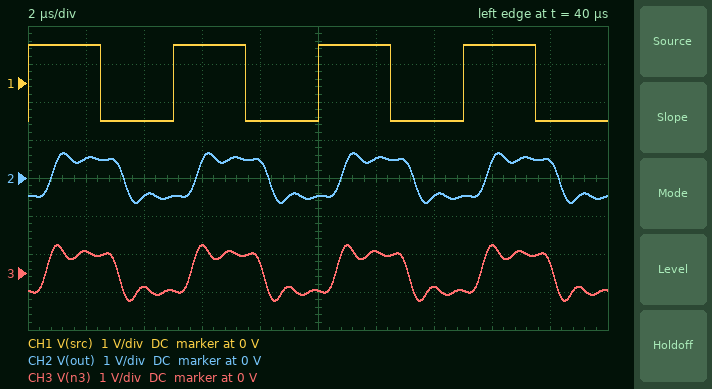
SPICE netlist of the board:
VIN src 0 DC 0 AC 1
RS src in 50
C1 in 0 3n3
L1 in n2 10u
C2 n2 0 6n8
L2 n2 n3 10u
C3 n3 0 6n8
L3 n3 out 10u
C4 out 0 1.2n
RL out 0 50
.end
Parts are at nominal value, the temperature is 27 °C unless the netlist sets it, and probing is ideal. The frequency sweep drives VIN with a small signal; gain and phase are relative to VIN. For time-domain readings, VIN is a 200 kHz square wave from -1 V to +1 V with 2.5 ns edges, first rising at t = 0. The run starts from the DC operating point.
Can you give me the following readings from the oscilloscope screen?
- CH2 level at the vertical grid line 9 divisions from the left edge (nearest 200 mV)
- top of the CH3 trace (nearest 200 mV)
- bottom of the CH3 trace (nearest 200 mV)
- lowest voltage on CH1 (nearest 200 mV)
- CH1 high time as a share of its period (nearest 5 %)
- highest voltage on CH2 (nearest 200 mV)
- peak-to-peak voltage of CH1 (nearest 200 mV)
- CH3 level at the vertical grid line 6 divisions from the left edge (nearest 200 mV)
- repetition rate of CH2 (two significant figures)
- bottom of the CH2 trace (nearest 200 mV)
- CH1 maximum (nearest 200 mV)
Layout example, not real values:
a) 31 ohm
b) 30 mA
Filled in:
a) 400 mV
b) 800 mV
c) -800 mV
d) -1.0 V
e) 50 %
f) 600 mV
g) 2.0 V
h) 600 mV
i) 200 kHz
j) -600 mV
k) 1.0 V
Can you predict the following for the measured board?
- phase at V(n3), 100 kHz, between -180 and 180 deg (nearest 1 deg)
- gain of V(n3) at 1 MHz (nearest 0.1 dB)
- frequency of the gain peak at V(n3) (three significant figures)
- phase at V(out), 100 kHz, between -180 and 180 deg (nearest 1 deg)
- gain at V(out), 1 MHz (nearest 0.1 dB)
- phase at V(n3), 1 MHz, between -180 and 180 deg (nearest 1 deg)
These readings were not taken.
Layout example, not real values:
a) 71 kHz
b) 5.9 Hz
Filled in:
a) -20 deg
b) -3.6 dB
c) 1.03 MHz
d) -27 deg
e) -6.3 dB
f) 120 deg
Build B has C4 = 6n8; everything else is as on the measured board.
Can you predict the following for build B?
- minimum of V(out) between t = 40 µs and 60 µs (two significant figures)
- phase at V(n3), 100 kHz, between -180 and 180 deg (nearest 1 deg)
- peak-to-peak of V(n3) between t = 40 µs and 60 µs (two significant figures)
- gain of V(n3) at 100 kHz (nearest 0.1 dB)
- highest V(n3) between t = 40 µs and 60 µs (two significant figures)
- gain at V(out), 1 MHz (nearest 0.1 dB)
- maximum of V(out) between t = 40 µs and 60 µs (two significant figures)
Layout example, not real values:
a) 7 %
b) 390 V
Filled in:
a) -640 mV
b) -24 deg
c) 1.3 V
d) -6.3 dB
e) 650 mV
f) -7.7 dB
g) 640 mV
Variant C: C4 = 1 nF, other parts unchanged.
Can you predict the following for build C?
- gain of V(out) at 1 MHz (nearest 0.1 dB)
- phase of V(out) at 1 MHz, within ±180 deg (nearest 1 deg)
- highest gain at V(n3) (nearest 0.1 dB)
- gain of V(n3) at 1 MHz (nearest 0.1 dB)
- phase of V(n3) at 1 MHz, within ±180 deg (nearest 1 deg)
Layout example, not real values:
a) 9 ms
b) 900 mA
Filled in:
a) -6.4 dB
b) 55 deg
c) -3.4 dB
d) -3.5 dB
e) 119 deg
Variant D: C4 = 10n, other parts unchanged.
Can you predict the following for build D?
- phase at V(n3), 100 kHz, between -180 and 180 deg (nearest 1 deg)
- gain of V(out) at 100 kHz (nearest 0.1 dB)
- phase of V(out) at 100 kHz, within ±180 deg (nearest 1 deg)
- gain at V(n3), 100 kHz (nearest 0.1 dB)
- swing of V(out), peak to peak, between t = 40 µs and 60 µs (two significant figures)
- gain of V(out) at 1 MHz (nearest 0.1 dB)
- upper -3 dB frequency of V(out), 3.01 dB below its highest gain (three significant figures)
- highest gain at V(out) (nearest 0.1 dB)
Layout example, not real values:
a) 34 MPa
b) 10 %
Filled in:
a) -27 deg
b) -6.2 dB
c) -34 deg
d) -6.5 dB
e) 1.2 V
f) -10.0 dB
g) 868 kHz
h) -6.0 dB
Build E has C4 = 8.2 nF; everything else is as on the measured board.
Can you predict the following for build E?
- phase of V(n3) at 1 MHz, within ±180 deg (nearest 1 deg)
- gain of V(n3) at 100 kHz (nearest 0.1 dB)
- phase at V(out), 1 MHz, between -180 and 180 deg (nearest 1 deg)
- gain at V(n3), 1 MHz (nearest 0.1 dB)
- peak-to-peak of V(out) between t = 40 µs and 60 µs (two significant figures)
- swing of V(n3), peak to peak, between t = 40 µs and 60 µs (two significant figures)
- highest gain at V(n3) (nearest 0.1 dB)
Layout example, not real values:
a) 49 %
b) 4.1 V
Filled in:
a) 146 deg
b) -6.4 dB
c) -4 deg
d) -0.5 dB
e) 1.2 V
f) 1.3 V
g) 2.0 dB
